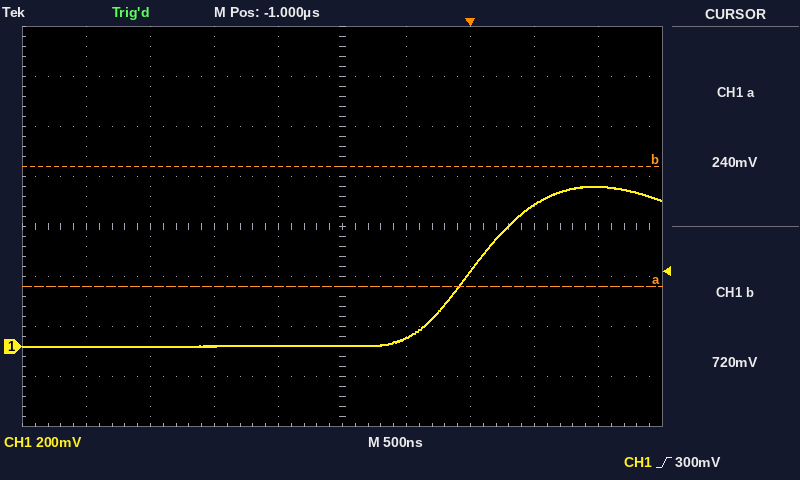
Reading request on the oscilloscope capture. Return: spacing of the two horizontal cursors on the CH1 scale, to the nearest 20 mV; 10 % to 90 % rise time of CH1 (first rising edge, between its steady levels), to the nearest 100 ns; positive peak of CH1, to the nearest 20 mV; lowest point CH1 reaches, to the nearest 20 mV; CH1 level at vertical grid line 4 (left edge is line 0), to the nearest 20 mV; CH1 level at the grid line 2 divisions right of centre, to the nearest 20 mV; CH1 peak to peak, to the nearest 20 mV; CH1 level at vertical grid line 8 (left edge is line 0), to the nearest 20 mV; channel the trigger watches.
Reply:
480 mV
900 ns
640 mV
0 mV
0 mV
300 mV
640 mV
560 mV
CH1
